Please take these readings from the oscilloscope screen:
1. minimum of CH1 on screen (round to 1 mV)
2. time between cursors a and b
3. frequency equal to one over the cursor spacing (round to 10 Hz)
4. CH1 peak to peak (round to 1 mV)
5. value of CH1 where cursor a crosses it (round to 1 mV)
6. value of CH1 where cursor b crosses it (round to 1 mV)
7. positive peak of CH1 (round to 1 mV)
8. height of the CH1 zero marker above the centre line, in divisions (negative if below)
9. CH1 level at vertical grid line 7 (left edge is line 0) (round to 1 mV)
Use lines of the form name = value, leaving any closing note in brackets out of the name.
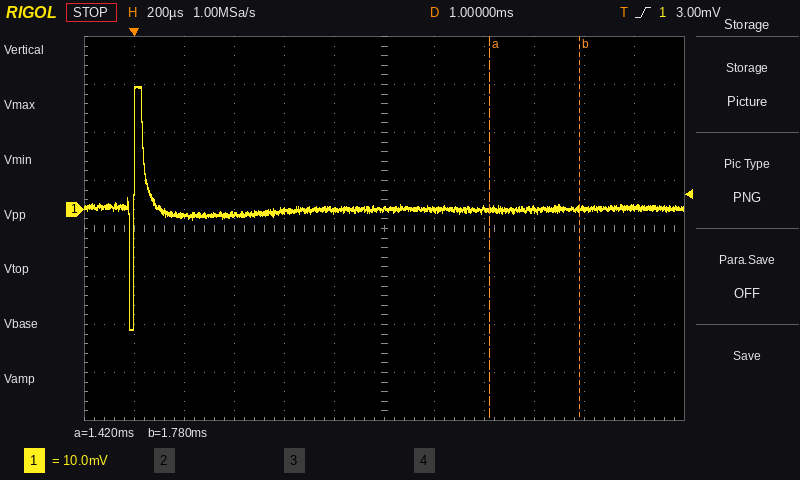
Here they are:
minimum of CH1 on screen = -25 mV
time between cursors a and b = 360 µs
frequency equal to one over the cursor spacing = 2.78 kHz
CH1 peak to peak = 51 mV
value of CH1 where cursor a crosses it = 0 mV
value of CH1 where cursor b crosses it = 0 mV
positive peak of CH1 = 26 mV
height of the CH1 zero marker above the centre line, in divisions = +0.4 div
CH1 level at vertical grid line 7 (left edge is line 0) = 0 mV
